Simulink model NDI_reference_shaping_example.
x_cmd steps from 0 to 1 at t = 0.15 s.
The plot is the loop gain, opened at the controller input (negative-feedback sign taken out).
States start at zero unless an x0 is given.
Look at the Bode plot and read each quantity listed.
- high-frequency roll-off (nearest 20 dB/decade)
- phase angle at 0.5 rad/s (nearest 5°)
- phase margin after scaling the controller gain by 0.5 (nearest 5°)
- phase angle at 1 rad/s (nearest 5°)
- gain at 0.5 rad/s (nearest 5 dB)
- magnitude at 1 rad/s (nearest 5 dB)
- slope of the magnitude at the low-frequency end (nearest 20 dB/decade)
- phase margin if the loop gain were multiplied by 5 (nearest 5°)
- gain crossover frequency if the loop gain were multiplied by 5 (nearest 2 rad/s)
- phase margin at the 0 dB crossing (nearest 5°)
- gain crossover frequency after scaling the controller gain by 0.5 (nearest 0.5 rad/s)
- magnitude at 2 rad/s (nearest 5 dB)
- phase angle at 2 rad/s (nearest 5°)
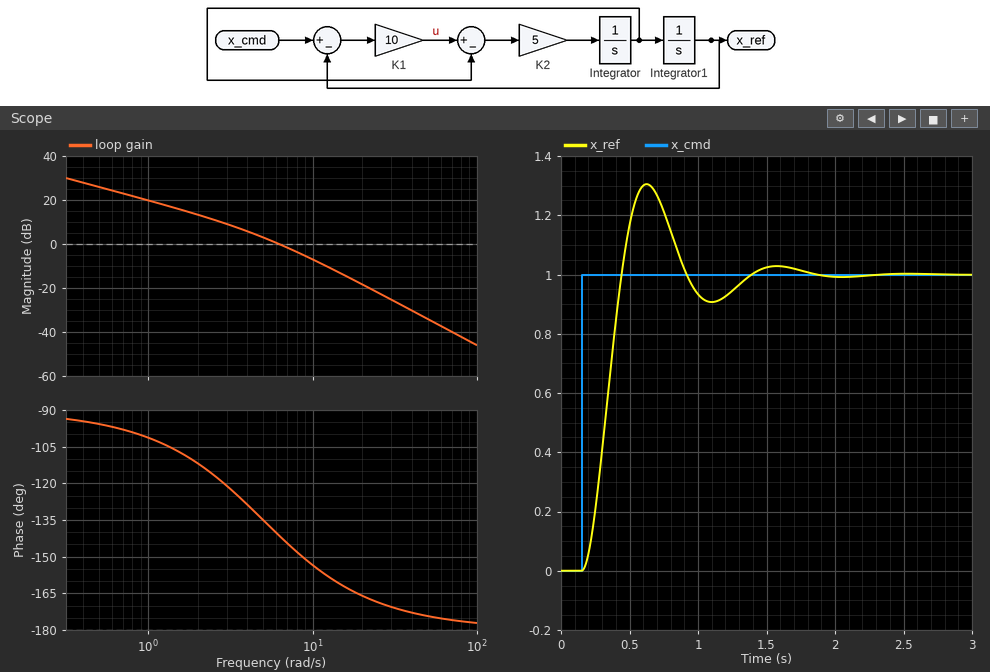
-40 dB/decade
-95°
50°
-100°
25 dB
20 dB
-20 dB/decade
20°
16 rad/s
40°
4.0 rad/s
15 dB
-110°
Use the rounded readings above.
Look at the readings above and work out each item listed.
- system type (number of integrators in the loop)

1
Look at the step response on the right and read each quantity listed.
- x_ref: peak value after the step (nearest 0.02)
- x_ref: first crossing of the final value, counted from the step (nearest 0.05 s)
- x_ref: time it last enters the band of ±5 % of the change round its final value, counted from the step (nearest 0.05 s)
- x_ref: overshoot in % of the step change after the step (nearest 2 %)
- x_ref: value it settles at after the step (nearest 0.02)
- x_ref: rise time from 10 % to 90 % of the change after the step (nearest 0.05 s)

1.30
0.30 s
1.10 s
30 %
1.00
0.20 s
